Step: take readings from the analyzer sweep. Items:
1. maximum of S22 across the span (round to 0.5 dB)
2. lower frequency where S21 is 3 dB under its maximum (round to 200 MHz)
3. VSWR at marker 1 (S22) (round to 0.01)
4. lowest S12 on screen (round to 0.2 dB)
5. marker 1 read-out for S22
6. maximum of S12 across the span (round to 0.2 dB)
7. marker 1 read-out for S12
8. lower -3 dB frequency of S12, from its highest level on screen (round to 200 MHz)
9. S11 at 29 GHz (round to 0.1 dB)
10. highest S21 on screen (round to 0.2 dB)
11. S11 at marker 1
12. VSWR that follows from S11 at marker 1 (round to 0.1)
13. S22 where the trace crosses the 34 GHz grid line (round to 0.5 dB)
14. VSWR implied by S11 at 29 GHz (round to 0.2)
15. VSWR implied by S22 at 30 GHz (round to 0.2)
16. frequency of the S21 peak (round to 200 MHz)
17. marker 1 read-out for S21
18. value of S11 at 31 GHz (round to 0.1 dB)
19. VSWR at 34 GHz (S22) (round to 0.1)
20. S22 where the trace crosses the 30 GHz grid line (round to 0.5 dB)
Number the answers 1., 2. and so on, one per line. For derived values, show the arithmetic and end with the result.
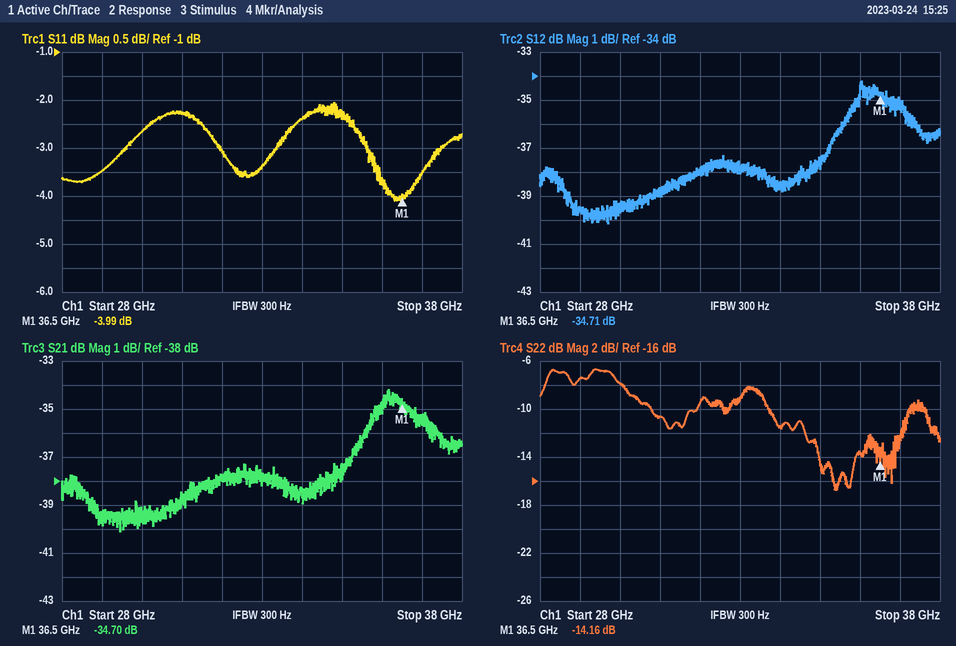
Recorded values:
1. -6.5 dB
2. 35.2 GHz
3. (1 + 0.1959)/(1 − 0.1959) ≈ 1.49
4. -40.2 dB
5. -14.16 dB
6. -34.2 dB
7. -34.71 dB
8. 35.2 GHz
9. -3.5 dB
10. -34.2 dB
11. -3.99 dB
12. (1 + 0.6317)/(1 − 0.6317) ≈ 4.4
13. -11.5 dB
14. |Γ| = 10^(-3.5/20) = 0.6683; VSWR = (1 + 0.6683)/(1 − 0.6683) ≈ 5.0
15. |Γ| = 10^(-8/20) = 0.3981; VSWR = (1 + 0.3981)/(1 − 0.3981) ≈ 2.32, so 2.4 to the nearest 0.2
16. 36.2 GHz
17. -34.70 dB
18. -2.3 dB
19. |Γ| = 10^(-11.5/20) = 0.2661; VSWR = (1 + 0.2661)/(1 − 0.2661) ≈ 1.7
20. -8.0 dB
